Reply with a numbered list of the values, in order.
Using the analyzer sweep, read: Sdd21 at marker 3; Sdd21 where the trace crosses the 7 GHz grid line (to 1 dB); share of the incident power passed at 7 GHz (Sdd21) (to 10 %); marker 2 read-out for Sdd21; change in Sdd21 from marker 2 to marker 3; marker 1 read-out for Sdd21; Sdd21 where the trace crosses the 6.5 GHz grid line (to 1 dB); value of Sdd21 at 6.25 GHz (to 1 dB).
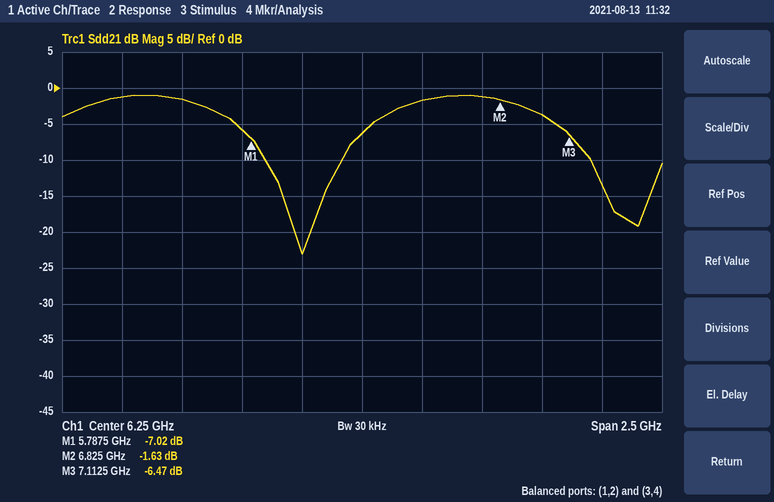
1. -6.47 dB
2. -4 dB
3. 40 %
4. -1.63 dB
5. -4.84 dB
6. -7.02 dB
7. -2 dB
8. -6 dB
